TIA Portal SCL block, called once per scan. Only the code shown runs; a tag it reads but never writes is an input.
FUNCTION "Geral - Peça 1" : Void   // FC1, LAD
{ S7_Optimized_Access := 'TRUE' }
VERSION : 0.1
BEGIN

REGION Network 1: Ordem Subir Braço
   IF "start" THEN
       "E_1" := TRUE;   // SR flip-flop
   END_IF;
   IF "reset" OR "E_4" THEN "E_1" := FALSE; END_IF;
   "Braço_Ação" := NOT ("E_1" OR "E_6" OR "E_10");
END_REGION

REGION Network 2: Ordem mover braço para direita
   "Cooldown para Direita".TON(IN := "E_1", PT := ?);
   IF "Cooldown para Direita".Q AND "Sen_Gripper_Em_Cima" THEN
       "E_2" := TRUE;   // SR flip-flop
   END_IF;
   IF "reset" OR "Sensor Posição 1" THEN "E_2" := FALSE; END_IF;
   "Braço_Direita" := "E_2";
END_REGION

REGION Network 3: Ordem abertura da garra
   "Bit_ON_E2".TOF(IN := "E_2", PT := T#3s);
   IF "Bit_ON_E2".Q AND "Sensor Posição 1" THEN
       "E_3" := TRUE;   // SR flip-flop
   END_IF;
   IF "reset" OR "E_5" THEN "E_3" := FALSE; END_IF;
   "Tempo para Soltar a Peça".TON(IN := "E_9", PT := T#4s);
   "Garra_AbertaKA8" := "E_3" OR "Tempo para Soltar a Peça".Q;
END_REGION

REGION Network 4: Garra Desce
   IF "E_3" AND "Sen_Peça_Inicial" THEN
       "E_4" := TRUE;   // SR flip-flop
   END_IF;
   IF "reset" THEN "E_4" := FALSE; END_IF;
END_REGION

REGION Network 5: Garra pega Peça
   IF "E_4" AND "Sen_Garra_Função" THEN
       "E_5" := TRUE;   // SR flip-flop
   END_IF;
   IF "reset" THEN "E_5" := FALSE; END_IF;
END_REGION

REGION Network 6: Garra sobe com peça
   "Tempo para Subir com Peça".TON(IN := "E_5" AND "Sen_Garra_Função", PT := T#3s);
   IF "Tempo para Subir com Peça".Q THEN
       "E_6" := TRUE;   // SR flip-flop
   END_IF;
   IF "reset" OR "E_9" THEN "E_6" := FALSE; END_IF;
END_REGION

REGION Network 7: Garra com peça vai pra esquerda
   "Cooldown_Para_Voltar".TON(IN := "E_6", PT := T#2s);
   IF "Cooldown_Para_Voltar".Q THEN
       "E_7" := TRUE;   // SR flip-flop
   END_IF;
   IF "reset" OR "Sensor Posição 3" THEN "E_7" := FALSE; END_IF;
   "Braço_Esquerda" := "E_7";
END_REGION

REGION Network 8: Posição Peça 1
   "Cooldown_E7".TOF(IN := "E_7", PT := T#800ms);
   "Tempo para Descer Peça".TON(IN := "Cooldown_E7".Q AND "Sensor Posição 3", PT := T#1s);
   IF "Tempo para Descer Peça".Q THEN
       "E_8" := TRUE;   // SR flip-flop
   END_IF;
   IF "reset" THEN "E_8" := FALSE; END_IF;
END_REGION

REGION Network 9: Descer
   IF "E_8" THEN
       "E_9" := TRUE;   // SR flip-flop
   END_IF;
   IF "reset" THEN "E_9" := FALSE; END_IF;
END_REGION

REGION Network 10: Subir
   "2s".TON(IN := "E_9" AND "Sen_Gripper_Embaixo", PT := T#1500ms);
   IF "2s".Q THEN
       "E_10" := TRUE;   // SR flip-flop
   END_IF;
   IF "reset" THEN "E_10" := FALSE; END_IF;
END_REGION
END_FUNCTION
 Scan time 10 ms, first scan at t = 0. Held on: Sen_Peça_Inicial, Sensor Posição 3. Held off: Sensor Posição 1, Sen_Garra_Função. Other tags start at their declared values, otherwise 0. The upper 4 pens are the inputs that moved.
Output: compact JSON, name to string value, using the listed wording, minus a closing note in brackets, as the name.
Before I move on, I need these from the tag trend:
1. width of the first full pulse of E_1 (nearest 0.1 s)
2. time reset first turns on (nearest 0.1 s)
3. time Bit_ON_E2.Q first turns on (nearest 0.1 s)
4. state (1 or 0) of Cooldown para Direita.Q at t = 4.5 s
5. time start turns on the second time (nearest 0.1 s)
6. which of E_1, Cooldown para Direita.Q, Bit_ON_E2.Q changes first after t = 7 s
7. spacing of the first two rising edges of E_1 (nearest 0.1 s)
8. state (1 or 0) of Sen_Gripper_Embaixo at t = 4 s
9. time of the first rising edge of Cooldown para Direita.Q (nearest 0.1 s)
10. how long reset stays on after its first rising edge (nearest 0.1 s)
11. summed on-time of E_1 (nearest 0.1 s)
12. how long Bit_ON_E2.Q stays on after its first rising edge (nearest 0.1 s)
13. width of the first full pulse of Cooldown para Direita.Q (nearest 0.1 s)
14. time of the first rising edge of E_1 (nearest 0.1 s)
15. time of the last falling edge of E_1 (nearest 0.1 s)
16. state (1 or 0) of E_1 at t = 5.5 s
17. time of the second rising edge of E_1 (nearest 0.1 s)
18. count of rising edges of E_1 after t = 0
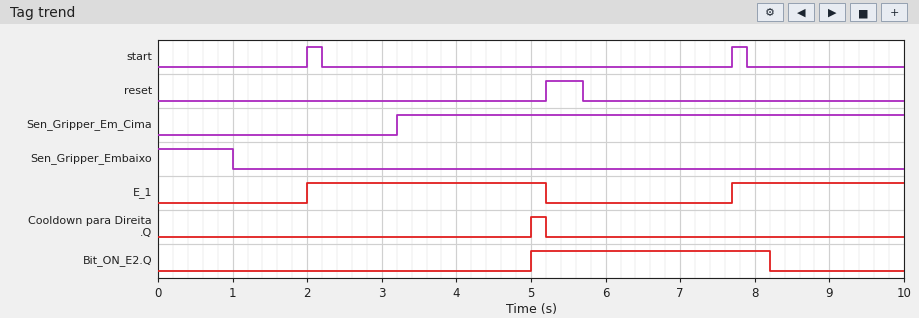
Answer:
{"width of the first full pulse of E_1": "3.2 s", "time reset first turns on": "5.2 s", "time Bit_ON_E2.Q first turns on": "5.0 s", "state (1 or 0) of Cooldown para Direita.Q at t = 4.5 s": "0", "time start turns on the second time": "7.7 s", "which of E_1, Cooldown para Direita.Q, Bit_ON_E2.Q changes first after t = 7 s": "E_1", "spacing of the first two rising edges of E_1": "5.7 s", "state (1 or 0) of Sen_Gripper_Embaixo at t = 4 s": "0", "time of the first rising edge of Cooldown para Direita.Q": "5.0 s", "how long reset stays on after its first rising edge": "0.5 s", "summed on-time of E_1": "5.5 s", "how long Bit_ON_E2.Q stays on after its first rising edge": "3.2 s", "width of the first full pulse of Cooldown para Direita.Q": "0.2 s", "time of the first rising edge of E_1": "2.0 s", "time of the last falling edge of E_1": "5.2 s", "state (1 or 0) of E_1 at t = 5.5 s": "0", "time of the second rising edge of E_1": "7.7 s", "count of rising edges of E_1 after t = 0": "2"}
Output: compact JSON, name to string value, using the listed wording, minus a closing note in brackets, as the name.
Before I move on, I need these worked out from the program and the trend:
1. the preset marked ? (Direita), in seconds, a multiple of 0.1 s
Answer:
{"the preset marked ? (Direita), in seconds, a multiple of 0.1 s": "3.0 s"}
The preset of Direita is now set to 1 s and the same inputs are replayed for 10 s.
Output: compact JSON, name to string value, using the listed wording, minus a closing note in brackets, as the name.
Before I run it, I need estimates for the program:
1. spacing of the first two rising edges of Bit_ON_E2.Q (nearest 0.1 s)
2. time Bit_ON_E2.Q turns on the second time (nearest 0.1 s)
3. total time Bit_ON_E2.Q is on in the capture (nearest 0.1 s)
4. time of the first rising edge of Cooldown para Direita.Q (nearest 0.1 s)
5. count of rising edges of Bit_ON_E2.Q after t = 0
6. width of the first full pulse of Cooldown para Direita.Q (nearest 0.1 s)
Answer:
{"spacing of the first two rising edges of Bit_ON_E2.Q": "5.5 s", "time Bit_ON_E2.Q turns on the second time": "8.7 s", "total time Bit_ON_E2.Q is on in the capture": "6.3 s", "time of the first rising edge of Cooldown para Direita.Q": "3.0 s", "count of rising edges of Bit_ON_E2.Q after t = 0": "2", "width of the first full pulse of Cooldown para Direita.Q": "2.2 s"}
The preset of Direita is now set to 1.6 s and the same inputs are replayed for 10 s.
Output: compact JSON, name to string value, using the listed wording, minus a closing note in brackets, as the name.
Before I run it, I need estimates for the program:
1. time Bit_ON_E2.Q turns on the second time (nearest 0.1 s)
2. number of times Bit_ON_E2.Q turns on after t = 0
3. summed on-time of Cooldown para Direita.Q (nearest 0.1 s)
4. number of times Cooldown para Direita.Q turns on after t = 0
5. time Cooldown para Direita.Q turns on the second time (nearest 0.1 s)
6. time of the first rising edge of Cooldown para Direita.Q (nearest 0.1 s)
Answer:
{"time Bit_ON_E2.Q turns on the second time": "9.3 s", "number of times Bit_ON_E2.Q turns on after t = 0": "2", "summed on-time of Cooldown para Direita.Q": "2.3 s", "number of times Cooldown para Direita.Q turns on after t = 0": "2", "time Cooldown para Direita.Q turns on the second time": "9.3 s", "time of the first rising edge of Cooldown para Direita.Q": "3.6 s"}
